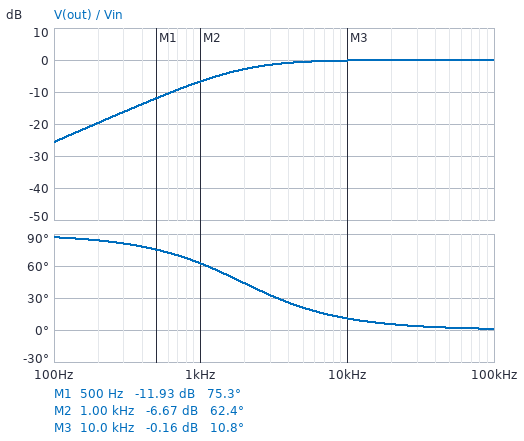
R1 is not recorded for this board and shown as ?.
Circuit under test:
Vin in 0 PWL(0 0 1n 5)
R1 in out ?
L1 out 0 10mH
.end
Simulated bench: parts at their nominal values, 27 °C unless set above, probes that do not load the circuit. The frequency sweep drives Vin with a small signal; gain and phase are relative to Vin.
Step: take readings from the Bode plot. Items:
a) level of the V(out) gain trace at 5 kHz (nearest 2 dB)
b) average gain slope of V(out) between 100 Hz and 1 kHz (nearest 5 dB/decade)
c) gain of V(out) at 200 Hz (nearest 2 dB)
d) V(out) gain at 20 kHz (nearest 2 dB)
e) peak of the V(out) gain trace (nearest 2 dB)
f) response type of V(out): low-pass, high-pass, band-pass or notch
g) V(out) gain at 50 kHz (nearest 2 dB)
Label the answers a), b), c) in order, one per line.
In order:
a) 0 dB
b) 20 dB/decade
c) -20 dB
d) 0 dB
e) 0 dB
f) high-pass
g) 0 dB
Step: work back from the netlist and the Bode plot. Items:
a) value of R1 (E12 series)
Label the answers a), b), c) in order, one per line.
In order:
a) 120 Ω
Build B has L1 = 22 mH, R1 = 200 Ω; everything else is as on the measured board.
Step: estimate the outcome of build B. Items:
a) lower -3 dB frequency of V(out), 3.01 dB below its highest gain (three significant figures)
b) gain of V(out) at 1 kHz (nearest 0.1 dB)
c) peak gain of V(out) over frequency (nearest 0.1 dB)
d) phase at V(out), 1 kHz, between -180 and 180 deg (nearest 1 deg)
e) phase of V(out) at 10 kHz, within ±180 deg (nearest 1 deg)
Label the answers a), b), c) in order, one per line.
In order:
a) 1.45 kHz
b) -4.9 dB
c) 0 dB
d) 55 deg
e) 8 deg
